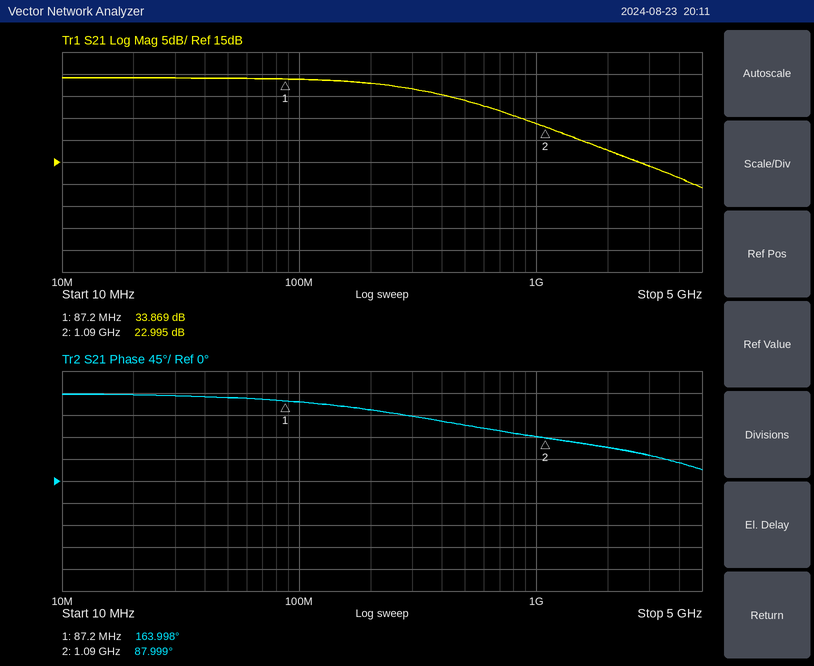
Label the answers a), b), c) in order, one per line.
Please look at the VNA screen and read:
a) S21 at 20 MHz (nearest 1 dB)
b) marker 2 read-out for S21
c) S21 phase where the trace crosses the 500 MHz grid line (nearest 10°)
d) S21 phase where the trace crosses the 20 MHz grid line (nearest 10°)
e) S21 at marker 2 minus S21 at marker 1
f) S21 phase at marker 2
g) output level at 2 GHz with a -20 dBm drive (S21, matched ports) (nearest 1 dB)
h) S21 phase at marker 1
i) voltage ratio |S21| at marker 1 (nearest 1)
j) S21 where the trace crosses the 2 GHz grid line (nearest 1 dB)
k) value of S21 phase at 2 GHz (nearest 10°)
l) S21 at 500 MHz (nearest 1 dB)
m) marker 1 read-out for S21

a) 34 dB
b) 22.995 dB
c) 110°
d) 180°
e) -10.874 dB
f) 87.999°
g) -2 dBm
h) 163.998°
i) 49
j) 18 dB
k) 70°
l) 29 dB
m) 33.869 dB
